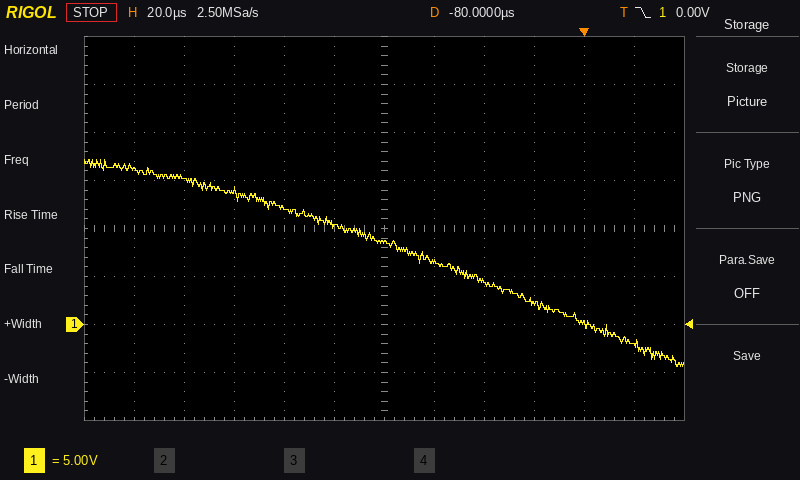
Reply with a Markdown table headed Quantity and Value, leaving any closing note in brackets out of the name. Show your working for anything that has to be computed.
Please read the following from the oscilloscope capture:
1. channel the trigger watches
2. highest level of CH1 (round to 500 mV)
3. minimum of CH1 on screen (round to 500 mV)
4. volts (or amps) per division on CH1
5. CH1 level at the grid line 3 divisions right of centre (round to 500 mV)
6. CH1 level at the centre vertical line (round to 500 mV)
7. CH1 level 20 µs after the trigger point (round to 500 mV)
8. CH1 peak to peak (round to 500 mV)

| Quantity | Value |
|---|---|
| channel the trigger watches | CH1 |
| highest level of CH1 | 17.0 V |
| minimum of CH1 on screen | -4.5 V |
| volts (or amps) per division on CH1 | 5 V |
| CH1 level at the grid line 3 divisions right of centre | 2.0 V |
| CH1 level at the centre vertical line | 8.5 V |
| CH1 level 20 µs after the trigger point | -2.0 V |
| CH1 peak to peak | 17.0 V − (-4.5 V) = 21.5 V |
